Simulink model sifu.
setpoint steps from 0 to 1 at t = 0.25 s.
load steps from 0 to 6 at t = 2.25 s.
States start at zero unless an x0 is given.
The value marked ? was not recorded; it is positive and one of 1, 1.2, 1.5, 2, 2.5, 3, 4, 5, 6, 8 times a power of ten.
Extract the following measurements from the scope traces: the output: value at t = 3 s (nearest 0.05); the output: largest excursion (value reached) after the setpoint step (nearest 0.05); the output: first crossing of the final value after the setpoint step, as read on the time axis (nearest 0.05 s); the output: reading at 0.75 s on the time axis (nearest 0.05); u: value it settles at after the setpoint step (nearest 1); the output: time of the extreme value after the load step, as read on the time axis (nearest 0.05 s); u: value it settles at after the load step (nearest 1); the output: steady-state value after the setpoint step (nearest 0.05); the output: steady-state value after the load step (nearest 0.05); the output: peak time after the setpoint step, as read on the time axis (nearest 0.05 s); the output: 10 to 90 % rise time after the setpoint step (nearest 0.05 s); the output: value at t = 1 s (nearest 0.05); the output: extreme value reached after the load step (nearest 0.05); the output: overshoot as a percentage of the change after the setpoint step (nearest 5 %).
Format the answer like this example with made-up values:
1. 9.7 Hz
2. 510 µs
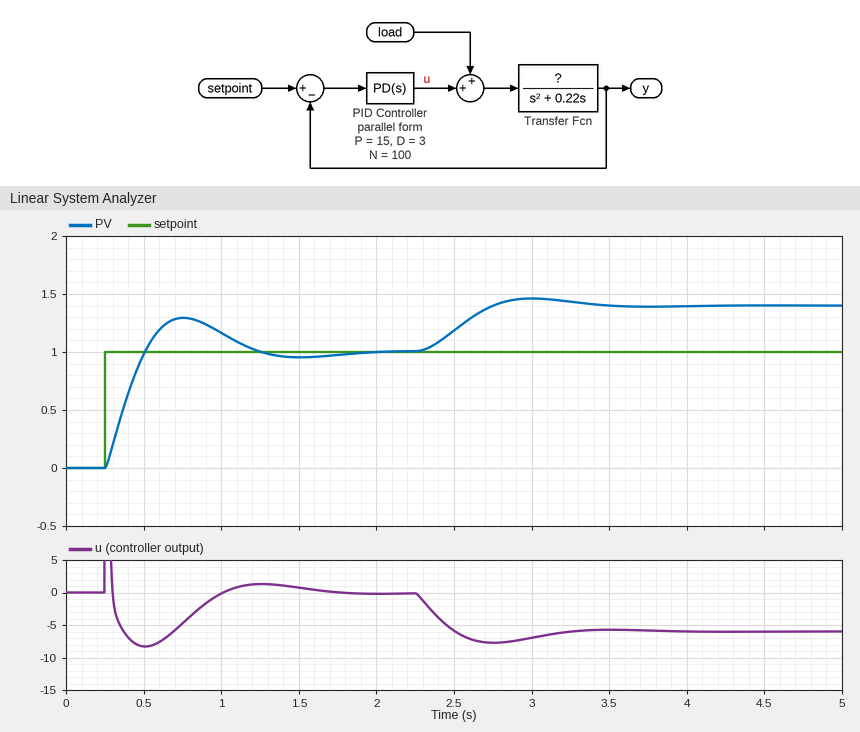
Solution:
1. 1.45
2. 1.30
3. 0.50 s
4. 1.30
5. 0
6. 3.00 s
7. -6
8. 1.00
9. 1.40
10. 0.75 s
11. 0.20 s
12. 1.15
13. 1.45
14. 30 %
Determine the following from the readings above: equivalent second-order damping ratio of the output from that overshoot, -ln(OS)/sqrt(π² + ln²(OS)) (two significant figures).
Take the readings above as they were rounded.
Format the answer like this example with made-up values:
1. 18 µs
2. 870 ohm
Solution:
1. 0.36
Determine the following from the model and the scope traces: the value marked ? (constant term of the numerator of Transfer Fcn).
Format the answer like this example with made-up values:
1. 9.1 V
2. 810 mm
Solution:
1. 1.5
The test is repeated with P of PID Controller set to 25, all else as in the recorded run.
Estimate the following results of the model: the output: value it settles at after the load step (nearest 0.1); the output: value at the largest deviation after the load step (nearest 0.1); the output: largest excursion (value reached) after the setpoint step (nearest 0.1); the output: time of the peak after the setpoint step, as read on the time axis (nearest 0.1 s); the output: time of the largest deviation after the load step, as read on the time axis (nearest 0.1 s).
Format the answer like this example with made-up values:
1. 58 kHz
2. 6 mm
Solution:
1. 1.2
2. 1.3
3. 1.4
4. 0.7 s
5. 2.8 s
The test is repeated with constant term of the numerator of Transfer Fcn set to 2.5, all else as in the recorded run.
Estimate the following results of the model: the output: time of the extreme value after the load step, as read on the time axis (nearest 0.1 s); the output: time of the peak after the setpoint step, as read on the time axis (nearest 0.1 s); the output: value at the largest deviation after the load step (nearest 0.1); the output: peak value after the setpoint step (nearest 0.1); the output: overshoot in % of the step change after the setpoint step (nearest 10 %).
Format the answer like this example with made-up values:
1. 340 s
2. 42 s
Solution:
1. 2.9 s
2. 0.6 s
3. 1.4
4. 1.2
5. 20 %
